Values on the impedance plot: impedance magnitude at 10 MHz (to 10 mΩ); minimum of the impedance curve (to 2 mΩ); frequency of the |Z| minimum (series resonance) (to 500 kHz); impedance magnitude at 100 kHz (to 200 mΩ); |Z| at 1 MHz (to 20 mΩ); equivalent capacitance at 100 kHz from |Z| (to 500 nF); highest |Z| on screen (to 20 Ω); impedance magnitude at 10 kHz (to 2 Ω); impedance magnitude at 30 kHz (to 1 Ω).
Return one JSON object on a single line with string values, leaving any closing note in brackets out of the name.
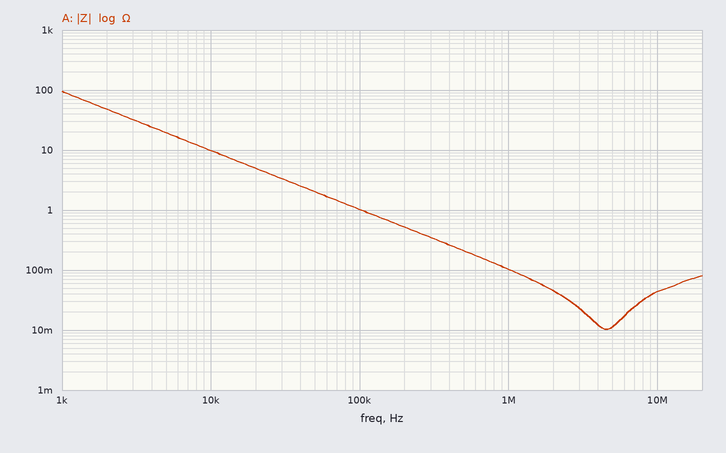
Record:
{"impedance magnitude at 10 MHz": "40 mΩ", "minimum of the impedance curve": "10 mΩ", "frequency of the |Z| minimum (series resonance)": "4.5 MHz", "impedance magnitude at 100 kHz": "1.0 Ω", "|Z| at 1 MHz": "100 mΩ", "equivalent capacitance at 100 kHz from |Z|": "1.5 µF", "highest |Z| on screen": "100 Ω", "impedance magnitude at 10 kHz": "10 Ω", "impedance magnitude at 30 kHz": "3 Ω"}
